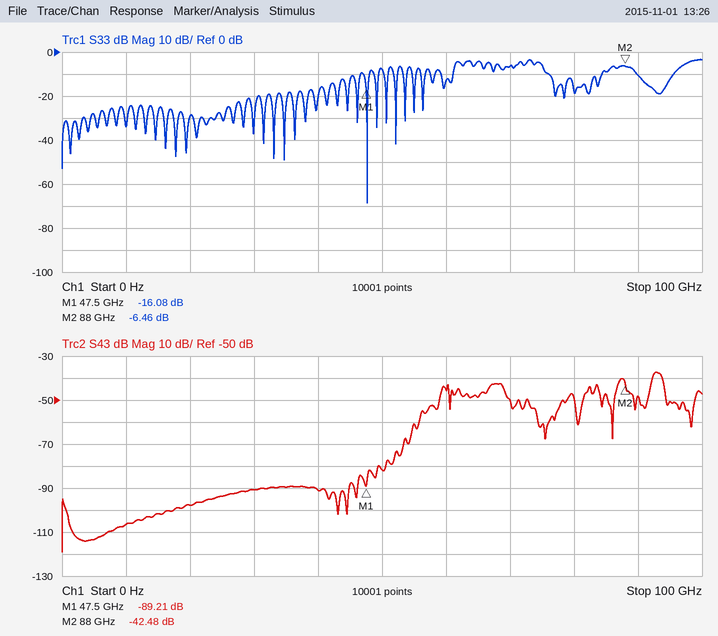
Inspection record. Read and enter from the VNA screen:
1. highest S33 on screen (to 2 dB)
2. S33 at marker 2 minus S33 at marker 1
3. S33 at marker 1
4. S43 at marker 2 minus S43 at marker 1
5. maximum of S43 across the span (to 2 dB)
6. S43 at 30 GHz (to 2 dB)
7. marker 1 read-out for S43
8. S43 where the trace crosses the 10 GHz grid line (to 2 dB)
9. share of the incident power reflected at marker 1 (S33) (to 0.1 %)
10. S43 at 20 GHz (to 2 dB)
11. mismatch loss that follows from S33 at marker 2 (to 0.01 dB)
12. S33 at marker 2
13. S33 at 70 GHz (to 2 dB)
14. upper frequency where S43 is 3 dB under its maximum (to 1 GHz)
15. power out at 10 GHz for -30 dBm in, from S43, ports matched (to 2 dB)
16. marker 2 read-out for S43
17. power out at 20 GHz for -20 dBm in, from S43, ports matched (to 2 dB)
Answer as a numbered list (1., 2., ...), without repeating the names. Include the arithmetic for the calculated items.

1. -4 dB
2. -6.46 − (-16.08) = 9.62 dB
3. -16.08 dB
4. -42.48 − (-89.21) = 46.73 dB
5. -38 dB
6. -90 dB
7. -89.21 dB
8. -106 dB
9. 10^(-16.08/10) ≈ 2.5 %
10. -98 dB
11. −10 log10(1 − 10^(-6.46/10)) ≈ 1.11 dB
12. -6.46 dB
13. -6 dB
14. 94 GHz
15. -30 dBm + (-106 dB) = -136 dBm
16. -42.48 dB
17. -20 dBm + (-98 dB) = -118 dBm
